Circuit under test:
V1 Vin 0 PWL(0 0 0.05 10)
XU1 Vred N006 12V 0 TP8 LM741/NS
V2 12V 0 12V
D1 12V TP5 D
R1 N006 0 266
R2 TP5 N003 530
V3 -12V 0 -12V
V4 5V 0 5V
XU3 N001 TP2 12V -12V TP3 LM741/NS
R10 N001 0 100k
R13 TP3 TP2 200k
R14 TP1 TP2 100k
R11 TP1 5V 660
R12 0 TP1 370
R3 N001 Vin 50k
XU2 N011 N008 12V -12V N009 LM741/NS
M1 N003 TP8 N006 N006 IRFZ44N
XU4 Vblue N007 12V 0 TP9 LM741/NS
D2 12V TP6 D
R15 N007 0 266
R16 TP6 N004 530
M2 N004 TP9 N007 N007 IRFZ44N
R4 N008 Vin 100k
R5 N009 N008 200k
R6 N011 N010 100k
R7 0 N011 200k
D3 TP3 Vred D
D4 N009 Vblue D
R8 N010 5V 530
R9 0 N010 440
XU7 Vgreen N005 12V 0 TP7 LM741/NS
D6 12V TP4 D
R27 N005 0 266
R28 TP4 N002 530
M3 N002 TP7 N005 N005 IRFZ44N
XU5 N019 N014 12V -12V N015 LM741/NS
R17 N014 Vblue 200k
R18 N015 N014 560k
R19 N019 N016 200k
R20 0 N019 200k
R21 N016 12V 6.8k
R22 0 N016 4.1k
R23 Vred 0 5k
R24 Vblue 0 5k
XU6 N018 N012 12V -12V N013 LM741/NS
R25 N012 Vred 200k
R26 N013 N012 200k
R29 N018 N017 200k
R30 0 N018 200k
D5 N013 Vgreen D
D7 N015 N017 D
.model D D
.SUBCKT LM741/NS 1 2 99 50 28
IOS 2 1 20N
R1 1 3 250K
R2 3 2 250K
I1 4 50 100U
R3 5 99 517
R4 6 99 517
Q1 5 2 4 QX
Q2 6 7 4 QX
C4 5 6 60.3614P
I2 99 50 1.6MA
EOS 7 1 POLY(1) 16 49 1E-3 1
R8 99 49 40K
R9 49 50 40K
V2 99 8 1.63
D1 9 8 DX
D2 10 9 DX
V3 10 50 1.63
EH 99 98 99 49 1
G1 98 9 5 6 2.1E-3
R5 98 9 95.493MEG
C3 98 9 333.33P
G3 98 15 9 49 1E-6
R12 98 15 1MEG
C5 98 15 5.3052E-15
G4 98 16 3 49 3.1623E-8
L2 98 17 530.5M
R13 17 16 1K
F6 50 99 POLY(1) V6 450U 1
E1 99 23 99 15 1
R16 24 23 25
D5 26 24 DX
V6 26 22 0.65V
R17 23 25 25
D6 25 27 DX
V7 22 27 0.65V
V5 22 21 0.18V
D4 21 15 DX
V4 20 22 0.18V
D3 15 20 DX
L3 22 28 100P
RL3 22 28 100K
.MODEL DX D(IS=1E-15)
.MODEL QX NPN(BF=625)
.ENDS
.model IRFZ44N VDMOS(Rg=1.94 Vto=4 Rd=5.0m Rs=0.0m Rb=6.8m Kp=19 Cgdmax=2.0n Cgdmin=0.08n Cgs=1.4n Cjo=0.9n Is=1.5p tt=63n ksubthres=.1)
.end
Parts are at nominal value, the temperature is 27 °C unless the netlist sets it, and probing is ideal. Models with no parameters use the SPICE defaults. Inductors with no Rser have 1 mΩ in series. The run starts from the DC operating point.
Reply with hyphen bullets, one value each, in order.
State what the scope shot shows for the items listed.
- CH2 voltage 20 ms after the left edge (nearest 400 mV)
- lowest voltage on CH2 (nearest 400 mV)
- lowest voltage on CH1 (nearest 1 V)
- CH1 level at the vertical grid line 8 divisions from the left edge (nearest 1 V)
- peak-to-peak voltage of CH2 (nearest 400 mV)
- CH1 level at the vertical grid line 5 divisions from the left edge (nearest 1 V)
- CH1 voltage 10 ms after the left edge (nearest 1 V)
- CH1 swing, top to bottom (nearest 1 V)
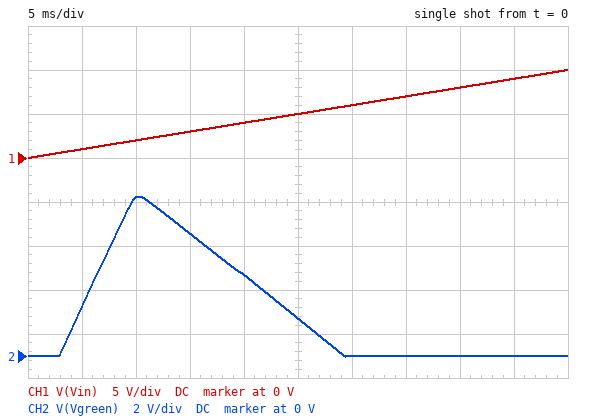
- 3.6 V
- 0 V
- 0 V
- 8 V
- 7.2 V
- 5 V
- 2 V
- 10 V
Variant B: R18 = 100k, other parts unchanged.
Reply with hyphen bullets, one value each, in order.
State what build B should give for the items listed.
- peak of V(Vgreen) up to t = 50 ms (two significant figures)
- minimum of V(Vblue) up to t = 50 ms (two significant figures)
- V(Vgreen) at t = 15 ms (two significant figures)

- 2.4 V
- 54 mV
- 630 mV
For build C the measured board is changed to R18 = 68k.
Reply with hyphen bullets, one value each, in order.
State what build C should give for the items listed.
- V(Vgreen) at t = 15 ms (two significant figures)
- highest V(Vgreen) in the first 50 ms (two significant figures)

- 280 mV
- 2.0 V
